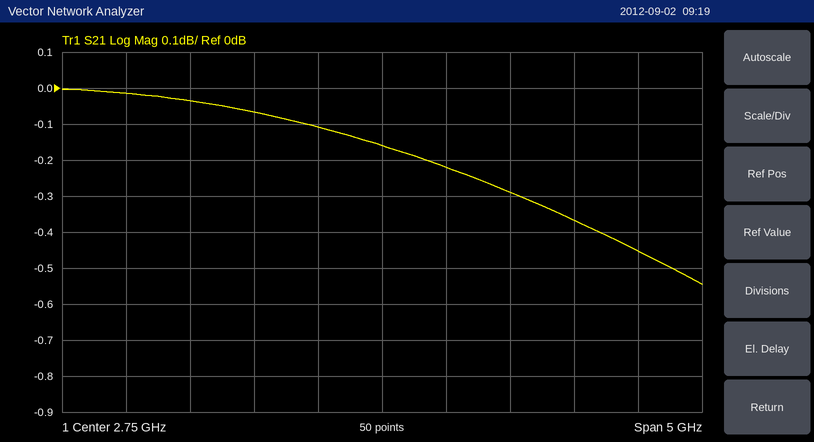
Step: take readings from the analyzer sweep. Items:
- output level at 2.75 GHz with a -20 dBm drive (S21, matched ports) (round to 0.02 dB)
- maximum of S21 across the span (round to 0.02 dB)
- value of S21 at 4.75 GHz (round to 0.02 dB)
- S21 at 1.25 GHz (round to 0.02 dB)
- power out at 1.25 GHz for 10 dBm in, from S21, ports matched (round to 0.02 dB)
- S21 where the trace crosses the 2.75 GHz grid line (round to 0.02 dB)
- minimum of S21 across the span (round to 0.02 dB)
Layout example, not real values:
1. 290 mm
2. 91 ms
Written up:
1. -20.16 dBm
2. 0.00 dB
3. -0.46 dB
4. -0.04 dB
5. 9.96 dBm
6. -0.16 dB
7. -0.54 dB
